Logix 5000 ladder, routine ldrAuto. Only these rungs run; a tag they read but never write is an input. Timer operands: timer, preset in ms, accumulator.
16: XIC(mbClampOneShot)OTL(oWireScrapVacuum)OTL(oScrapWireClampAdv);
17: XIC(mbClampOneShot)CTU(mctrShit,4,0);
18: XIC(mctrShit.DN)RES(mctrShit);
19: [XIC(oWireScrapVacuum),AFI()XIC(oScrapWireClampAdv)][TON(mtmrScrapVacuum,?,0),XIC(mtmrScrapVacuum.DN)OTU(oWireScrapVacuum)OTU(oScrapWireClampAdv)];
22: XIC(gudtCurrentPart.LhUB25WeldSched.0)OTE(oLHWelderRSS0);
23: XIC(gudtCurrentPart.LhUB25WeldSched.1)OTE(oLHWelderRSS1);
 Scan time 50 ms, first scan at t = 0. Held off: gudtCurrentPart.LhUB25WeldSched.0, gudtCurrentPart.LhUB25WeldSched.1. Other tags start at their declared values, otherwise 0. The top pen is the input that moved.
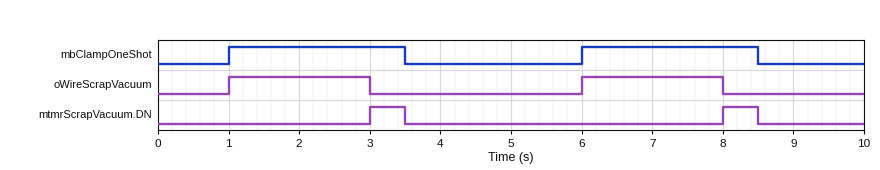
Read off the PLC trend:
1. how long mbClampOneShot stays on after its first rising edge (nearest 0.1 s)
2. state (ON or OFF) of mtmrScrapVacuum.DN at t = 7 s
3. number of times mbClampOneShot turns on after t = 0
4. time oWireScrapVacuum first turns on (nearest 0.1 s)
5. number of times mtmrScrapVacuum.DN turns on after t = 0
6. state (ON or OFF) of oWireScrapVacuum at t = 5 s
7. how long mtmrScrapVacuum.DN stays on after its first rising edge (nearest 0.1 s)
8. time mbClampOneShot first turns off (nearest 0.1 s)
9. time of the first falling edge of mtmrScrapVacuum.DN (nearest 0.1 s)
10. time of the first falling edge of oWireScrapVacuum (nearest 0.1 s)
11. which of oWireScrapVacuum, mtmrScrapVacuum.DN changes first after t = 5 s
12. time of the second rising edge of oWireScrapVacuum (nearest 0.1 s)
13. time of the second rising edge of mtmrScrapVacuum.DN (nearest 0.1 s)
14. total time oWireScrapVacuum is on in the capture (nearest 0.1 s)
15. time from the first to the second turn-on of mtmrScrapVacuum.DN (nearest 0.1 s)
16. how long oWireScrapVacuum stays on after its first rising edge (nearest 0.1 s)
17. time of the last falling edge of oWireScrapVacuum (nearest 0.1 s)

2.5 s
OFF
2
1.0 s
2
OFF
0.5 s
3.5 s
3.5 s
3.0 s
oWireScrapVacuum
6.0 s
8.0 s
4.0 s
5.0 s
2.0 s
8.0 s
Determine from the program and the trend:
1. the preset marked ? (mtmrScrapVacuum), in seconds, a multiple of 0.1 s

2.0 s
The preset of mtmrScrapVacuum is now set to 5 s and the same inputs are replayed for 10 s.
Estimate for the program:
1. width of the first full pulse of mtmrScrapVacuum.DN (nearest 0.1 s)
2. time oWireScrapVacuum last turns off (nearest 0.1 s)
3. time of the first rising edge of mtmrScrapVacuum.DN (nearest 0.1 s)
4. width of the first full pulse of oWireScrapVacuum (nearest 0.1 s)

2.5 s
6.0 s
6.0 s
5.0 s
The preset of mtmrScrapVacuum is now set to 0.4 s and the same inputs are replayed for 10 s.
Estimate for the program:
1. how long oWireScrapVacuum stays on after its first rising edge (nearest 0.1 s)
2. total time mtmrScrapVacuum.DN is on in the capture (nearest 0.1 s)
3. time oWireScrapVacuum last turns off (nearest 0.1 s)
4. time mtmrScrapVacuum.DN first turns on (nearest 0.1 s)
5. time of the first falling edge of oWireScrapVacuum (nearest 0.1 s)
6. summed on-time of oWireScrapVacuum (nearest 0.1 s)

0.4 s
4.2 s
6.4 s
1.4 s
1.4 s
0.8 s
